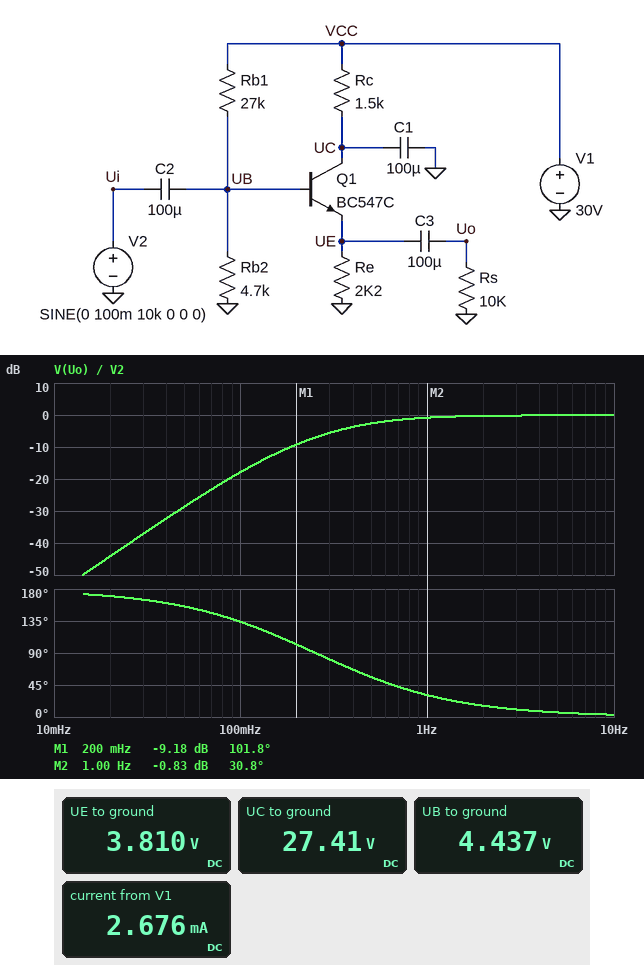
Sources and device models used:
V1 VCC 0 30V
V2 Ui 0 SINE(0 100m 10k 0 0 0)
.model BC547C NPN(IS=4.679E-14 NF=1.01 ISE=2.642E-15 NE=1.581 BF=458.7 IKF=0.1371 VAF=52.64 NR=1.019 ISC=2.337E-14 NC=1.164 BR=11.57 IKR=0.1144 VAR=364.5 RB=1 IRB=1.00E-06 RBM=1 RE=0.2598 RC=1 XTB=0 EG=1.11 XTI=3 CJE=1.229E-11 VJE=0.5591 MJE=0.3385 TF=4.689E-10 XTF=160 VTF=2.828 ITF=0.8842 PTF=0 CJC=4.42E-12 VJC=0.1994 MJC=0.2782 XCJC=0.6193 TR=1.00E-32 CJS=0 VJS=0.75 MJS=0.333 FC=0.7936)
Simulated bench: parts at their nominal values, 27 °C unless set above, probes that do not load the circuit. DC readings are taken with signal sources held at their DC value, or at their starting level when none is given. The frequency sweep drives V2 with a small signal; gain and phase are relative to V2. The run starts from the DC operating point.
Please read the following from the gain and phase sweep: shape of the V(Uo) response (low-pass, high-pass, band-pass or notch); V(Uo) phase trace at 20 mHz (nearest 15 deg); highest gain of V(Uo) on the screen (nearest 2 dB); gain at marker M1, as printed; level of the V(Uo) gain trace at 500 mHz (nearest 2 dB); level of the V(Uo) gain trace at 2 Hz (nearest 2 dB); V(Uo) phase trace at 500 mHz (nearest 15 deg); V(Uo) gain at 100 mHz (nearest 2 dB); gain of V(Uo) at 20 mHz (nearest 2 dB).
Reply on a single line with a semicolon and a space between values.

high-pass; 165 deg; 0 dB; -9.18 dB; -2 dB; 0 dB; 60 deg; -18 dB; -44 dB
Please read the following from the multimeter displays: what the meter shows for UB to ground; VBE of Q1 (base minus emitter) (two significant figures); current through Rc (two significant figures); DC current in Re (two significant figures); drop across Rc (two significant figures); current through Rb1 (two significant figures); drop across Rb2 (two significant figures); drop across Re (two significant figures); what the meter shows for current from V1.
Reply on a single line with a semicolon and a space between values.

4.437 V; 630 mV; 1.7 mA; 1.7 mA; 2.6 V; 950 µA; 4.4 V; 3.8 V; 2.676 mA
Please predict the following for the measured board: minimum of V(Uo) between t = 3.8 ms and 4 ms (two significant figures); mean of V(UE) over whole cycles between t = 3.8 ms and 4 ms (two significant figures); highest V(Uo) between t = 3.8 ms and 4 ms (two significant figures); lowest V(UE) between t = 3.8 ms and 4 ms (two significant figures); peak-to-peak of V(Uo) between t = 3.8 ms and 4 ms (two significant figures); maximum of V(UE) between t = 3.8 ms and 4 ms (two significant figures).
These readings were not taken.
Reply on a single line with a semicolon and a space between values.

-99 mV; 3.8 V; 99 mV; 3.7 V; 200 mV; 3.9 V
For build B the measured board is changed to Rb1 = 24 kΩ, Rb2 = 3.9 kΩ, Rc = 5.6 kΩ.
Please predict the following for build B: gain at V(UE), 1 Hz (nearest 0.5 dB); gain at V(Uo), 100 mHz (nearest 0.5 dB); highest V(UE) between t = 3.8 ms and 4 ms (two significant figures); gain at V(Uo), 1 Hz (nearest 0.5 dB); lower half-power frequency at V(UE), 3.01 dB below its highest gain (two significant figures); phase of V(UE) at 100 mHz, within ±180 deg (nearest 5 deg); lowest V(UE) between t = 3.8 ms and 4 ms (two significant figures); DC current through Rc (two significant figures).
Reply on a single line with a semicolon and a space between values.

-1.0 dB; -19.5 dB; 3.7 V; -1.0 dB; 480 mHz; 80 deg; 3.5 V; 1.6 mA
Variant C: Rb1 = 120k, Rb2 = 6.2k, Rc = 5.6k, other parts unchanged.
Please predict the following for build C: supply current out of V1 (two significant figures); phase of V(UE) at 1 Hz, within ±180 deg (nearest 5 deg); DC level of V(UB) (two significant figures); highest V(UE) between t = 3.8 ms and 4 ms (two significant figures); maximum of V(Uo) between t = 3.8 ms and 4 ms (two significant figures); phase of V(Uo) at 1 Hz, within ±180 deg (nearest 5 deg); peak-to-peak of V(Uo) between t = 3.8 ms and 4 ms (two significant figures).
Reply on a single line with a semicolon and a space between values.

640 µA; 15 deg; 1.5 V; 980 mV; 97 mV; 25 deg; 190 mV
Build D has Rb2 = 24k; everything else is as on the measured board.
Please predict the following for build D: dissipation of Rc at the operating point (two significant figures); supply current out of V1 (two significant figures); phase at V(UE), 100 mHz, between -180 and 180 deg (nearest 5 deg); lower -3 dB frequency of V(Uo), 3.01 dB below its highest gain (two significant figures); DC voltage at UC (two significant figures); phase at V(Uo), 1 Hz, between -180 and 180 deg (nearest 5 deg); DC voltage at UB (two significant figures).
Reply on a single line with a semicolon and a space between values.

55 mW; 6.6 mA; 50 deg; 220 mHz; 21 V; 15 deg; 14 V
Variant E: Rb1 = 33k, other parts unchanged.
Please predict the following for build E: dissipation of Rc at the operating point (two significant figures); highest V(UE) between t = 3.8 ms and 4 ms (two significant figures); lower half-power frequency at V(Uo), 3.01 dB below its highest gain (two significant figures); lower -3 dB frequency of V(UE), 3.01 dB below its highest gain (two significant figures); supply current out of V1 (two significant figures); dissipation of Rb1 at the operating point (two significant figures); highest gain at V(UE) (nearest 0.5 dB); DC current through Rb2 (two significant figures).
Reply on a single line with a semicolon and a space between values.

3.0 mW; 3.2 V; 440 mHz; 390 mHz; 2.2 mA; 21 mW; 0 dB; 790 µA
